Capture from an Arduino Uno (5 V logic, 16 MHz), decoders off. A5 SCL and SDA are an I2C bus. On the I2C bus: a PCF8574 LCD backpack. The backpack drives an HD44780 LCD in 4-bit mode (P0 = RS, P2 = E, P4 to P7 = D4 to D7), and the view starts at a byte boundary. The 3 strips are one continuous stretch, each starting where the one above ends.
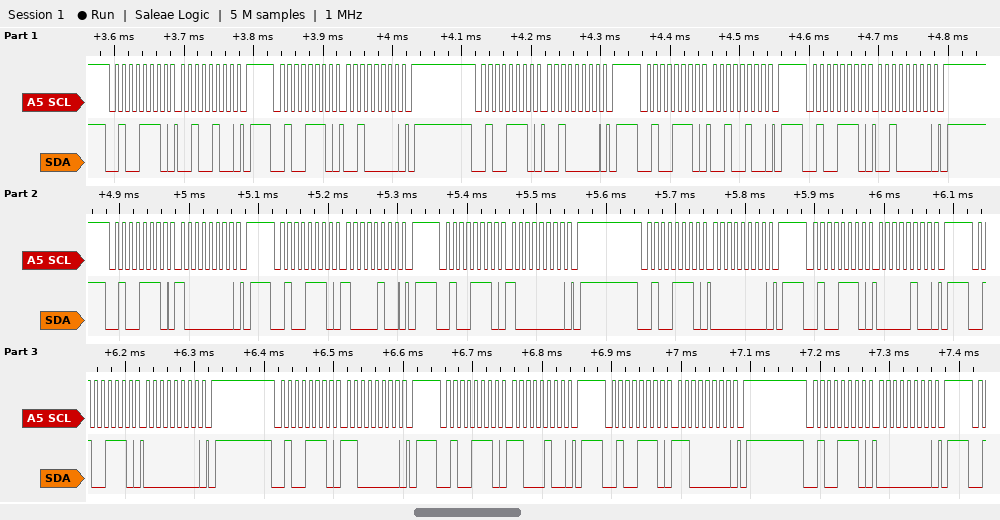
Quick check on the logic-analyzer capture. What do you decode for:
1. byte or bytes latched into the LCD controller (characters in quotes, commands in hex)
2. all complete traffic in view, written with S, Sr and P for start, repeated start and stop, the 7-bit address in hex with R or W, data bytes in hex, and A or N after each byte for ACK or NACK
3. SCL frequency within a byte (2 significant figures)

0x28 0x0C
S 27W A 24 A P S 27W A 20 A P S 27W A 20 A P S 27W A 24 A P S 27W A 20 A P S 27W A 80 A P S 27W A 84 A P S 27W A 80 A P S 27W A 00 A P S 27W A 04 A P S 27W A 00 A P S 27W A C0 A P S 27W A C4 A P S 27W A C0 A P S 27W A 00 A P
100 kHz
